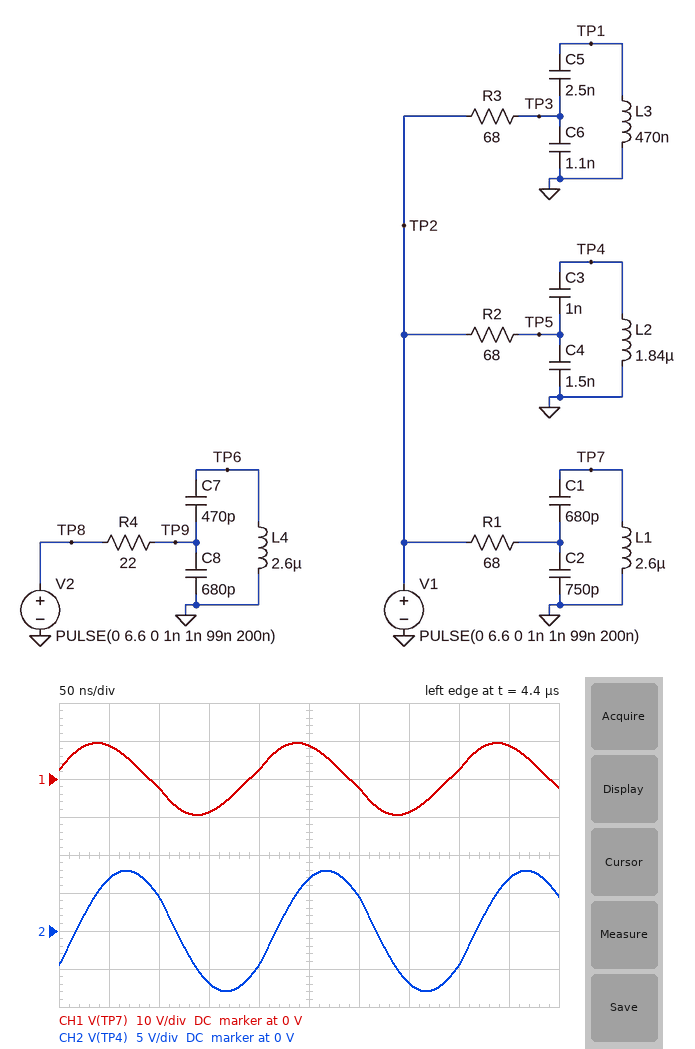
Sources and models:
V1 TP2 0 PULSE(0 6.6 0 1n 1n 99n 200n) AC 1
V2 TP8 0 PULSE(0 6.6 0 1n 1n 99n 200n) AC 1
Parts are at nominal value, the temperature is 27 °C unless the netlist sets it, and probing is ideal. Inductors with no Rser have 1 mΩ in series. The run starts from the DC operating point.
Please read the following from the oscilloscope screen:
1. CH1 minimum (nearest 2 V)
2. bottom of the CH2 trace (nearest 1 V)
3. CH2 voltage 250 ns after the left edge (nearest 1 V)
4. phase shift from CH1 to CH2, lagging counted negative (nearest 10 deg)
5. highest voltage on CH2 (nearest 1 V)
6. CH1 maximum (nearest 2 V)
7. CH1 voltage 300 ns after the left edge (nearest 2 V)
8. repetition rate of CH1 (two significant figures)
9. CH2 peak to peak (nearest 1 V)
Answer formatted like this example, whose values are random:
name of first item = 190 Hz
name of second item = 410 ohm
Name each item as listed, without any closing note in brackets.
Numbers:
CH1 minimum = -10 V
bottom of the CH2 trace = -8 V
CH2 voltage 250 ns after the left edge = 7 V
phase shift from CH1 to CH2, lagging counted negative = -50 deg
highest voltage on CH2 = 8 V
CH1 maximum = 10 V
CH1 voltage 300 ns after the left edge = -2 V
repetition rate of CH1 = 5.0 MHz
CH2 peak to peak = 16 V
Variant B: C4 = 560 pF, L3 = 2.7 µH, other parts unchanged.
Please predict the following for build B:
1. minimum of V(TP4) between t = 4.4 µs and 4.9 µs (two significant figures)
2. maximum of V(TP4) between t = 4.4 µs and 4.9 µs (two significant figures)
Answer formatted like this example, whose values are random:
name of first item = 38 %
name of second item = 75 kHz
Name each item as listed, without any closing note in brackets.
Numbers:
minimum of V(TP4) between t = 4.4 µs and 4.9 µs = -5.8 V
maximum of V(TP4) between t = 4.4 µs and 4.9 µs = 5.8 V
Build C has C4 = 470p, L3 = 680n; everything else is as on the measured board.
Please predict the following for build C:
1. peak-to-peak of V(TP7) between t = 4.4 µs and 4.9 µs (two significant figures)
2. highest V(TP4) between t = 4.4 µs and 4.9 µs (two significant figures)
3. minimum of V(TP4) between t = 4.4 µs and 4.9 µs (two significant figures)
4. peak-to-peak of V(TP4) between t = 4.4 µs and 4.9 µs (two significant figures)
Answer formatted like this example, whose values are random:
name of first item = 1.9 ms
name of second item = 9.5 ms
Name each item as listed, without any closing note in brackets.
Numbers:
peak-to-peak of V(TP7) between t = 4.4 µs and 4.9 µs = 19 V
highest V(TP4) between t = 4.4 µs and 4.9 µs = 5.4 V
minimum of V(TP4) between t = 4.4 µs and 4.9 µs = -5.4 V
peak-to-peak of V(TP4) between t = 4.4 µs and 4.9 µs = 11 V
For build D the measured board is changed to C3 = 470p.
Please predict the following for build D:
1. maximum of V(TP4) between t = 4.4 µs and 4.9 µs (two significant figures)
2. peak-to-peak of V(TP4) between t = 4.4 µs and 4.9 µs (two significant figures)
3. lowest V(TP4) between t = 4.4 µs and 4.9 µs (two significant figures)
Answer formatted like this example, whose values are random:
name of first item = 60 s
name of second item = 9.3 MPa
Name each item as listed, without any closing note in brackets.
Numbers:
maximum of V(TP4) between t = 4.4 µs and 4.9 µs = 2.3 V
peak-to-peak of V(TP4) between t = 4.4 µs and 4.9 µs = 4.6 V
lowest V(TP4) between t = 4.4 µs and 4.9 µs = -2.3 V
